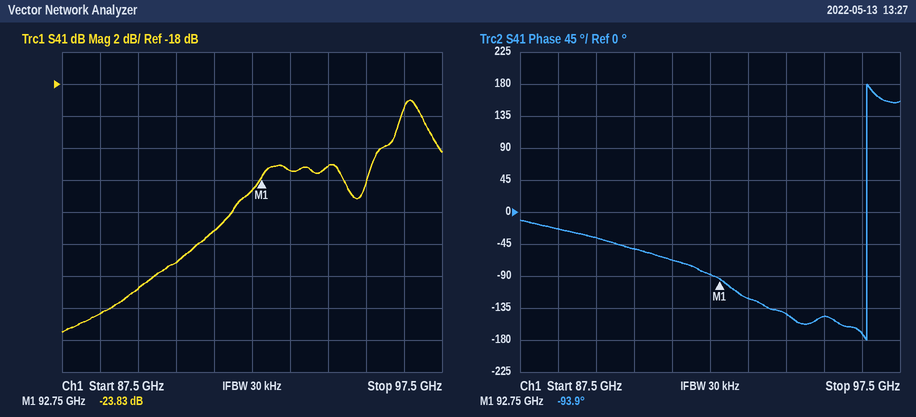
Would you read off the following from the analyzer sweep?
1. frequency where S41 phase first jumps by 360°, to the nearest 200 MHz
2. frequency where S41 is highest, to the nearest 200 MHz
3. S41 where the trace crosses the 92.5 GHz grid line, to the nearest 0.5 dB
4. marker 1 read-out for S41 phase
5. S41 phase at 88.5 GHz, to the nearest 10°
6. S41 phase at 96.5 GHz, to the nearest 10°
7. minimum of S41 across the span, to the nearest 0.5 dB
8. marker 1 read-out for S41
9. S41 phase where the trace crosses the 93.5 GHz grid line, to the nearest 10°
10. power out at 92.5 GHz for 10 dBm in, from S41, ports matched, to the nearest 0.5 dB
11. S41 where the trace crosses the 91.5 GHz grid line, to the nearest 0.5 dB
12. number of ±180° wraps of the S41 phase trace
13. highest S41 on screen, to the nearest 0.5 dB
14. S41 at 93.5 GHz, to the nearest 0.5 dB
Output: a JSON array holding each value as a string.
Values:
["96.6 GHz", "96.6 GHz", "-24.5 dB", "-93.9°", "-20°", "-170°", "-33.5 dB", "-23.83 dB", "-120°", "-14.5 dBm", "-27.0 dB", "1", "-19.0 dB", "-23.5 dB"]
